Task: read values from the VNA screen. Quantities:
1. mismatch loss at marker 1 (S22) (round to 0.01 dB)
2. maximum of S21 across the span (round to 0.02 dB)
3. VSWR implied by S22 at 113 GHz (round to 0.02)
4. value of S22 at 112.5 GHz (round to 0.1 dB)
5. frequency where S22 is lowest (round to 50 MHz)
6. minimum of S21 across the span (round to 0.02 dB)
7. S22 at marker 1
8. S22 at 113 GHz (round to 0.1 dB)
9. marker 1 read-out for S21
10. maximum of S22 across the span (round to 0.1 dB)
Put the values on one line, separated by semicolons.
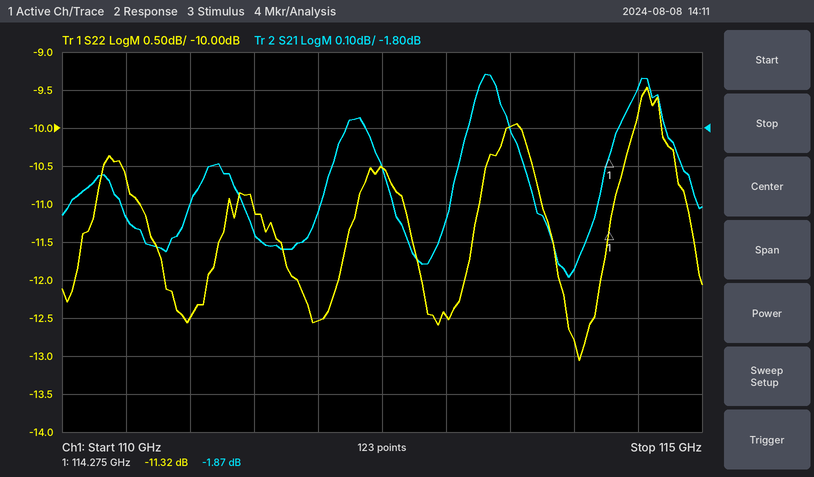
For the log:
0.33 dB; -1.66 dB; 1.62; -10.5 dB; 114.05 GHz; -2.20 dB; -11.32 dB; -12.5 dB; -1.87 dB; -9.5 dB
